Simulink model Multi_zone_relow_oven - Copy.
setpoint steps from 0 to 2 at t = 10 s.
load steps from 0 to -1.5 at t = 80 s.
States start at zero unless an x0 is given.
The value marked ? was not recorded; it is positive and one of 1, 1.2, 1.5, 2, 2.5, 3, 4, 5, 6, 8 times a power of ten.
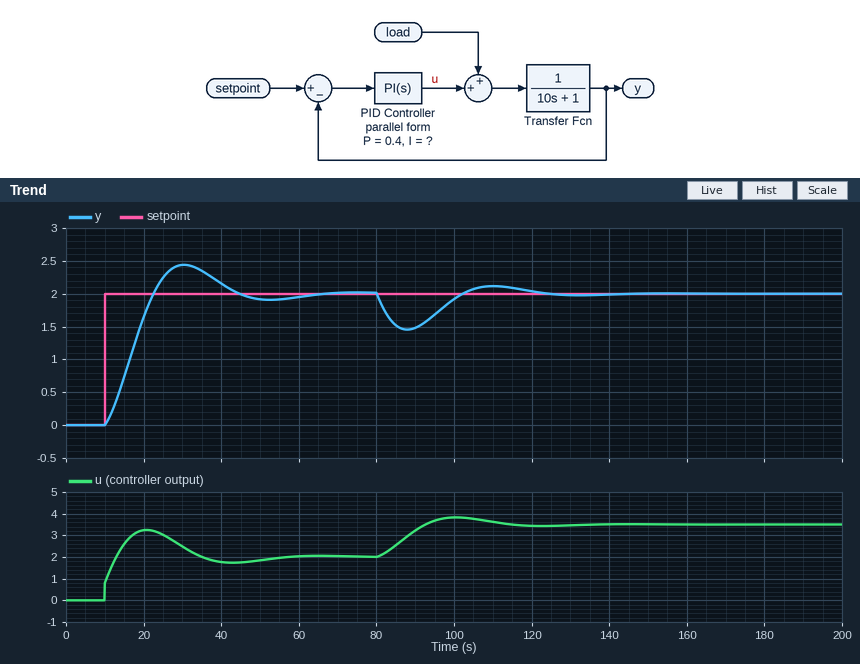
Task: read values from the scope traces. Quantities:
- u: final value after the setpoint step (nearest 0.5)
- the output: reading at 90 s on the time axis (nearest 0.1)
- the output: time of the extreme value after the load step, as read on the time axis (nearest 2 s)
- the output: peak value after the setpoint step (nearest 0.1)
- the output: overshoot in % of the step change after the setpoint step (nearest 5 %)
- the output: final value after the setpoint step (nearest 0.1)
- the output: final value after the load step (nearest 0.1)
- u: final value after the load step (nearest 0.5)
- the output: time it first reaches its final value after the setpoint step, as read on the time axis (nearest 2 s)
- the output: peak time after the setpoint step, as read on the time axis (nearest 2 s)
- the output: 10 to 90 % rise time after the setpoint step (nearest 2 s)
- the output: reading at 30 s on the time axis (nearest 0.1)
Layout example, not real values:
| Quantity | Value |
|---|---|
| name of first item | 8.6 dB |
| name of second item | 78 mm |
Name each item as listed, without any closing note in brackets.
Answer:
| Quantity | Value |
|---|---|
| u: final value after the setpoint step | 2.0 |
| the output: reading at 90 s on the time axis | 1.5 |
| the output: time of the extreme value after the load step, as read on the time axis | 88 s |
| the output: peak value after the setpoint step | 2.4 |
| the output: overshoot in % of the step change after the setpoint step | 20 % |
| the output: final value after the setpoint step | 2.0 |
| the output: final value after the load step | 2.0 |
| u: final value after the load step | 3.5 |
| the output: time it first reaches its final value after the setpoint step, as read on the time axis | 22 s |
| the output: peak time after the setpoint step, as read on the time axis | 30 s |
| the output: 10 to 90 % rise time after the setpoint step | 10 s |
| the output: reading at 30 s on the time axis | 2.4 |
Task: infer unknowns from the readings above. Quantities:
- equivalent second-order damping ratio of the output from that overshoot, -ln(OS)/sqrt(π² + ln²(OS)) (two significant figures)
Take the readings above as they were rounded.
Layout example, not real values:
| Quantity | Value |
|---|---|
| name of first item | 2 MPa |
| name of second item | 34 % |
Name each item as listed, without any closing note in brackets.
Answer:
| Quantity | Value |
|---|---|
| equivalent second-order damping ratio of the output from that overshoot, -ln(OS)/sqrt(π² + ln²(OS)) | 0.46 |
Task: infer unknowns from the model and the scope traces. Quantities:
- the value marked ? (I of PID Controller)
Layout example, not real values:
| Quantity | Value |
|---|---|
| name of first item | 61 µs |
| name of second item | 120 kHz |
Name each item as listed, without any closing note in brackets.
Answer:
| Quantity | Value |
|---|---|
| the value marked ? | 0.25 |
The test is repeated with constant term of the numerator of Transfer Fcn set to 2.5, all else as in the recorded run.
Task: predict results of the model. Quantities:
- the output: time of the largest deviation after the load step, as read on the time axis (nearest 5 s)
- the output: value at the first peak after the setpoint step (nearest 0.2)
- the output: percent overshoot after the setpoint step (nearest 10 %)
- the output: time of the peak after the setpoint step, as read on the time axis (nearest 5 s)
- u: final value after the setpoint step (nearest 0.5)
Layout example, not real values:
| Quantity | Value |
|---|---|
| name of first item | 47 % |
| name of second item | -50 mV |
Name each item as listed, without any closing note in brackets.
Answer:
| Quantity | Value |
|---|---|
| the output: time of the largest deviation after the load step, as read on the time axis | 85 s |
| the output: value at the first peak after the setpoint step | 2.6 |
| the output: percent overshoot after the setpoint step | 30 % |
| the output: time of the peak after the setpoint step, as read on the time axis | 20 s |
| u: final value after the setpoint step | 1.0 |
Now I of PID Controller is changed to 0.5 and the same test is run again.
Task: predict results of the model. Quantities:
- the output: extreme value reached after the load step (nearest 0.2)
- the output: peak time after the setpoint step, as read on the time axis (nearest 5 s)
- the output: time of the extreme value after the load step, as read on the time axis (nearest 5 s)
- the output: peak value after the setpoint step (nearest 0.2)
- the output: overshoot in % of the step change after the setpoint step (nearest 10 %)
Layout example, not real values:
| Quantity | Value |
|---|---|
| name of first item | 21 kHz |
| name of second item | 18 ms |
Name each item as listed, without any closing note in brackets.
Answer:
| Quantity | Value |
|---|---|
| the output: extreme value reached after the load step | 1.6 |
| the output: peak time after the setpoint step, as read on the time axis | 25 s |
| the output: time of the extreme value after the load step, as read on the time axis | 85 s |
| the output: peak value after the setpoint step | 2.8 |
| the output: overshoot in % of the step change after the setpoint step | 40 % |
